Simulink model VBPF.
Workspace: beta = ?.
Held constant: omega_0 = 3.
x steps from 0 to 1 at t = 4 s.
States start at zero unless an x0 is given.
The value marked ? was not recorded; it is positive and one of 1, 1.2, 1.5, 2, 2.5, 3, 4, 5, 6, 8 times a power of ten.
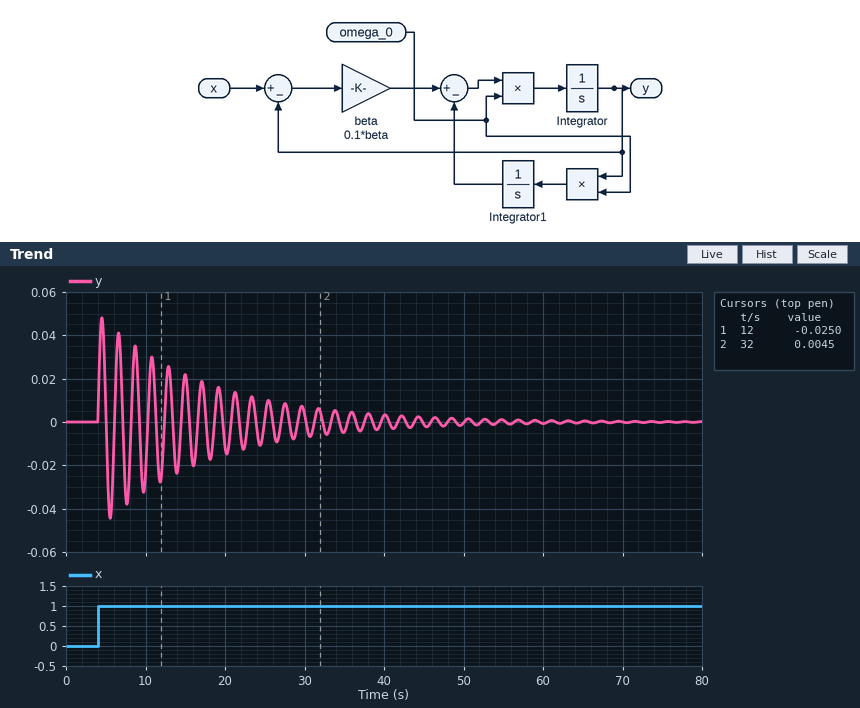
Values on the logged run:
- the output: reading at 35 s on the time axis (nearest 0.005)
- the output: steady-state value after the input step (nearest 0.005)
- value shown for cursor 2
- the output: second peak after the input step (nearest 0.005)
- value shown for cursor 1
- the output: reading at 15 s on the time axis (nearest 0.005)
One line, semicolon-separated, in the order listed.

-0.005; 0.000; 0.0045; 0.040; -0.0250; 0.020
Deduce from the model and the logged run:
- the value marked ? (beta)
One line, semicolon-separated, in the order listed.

0.5
